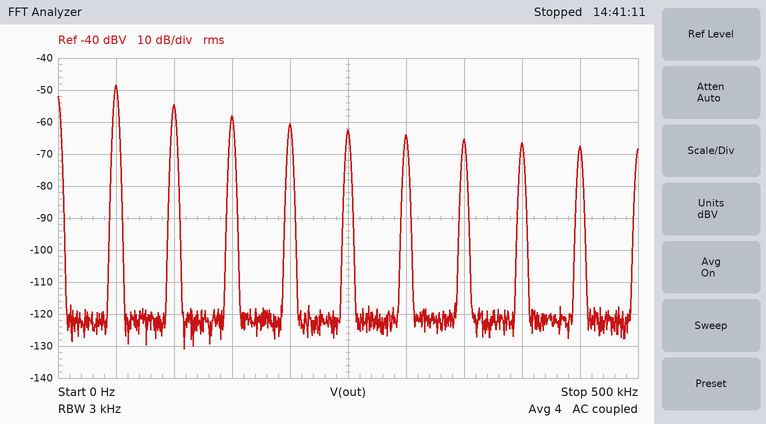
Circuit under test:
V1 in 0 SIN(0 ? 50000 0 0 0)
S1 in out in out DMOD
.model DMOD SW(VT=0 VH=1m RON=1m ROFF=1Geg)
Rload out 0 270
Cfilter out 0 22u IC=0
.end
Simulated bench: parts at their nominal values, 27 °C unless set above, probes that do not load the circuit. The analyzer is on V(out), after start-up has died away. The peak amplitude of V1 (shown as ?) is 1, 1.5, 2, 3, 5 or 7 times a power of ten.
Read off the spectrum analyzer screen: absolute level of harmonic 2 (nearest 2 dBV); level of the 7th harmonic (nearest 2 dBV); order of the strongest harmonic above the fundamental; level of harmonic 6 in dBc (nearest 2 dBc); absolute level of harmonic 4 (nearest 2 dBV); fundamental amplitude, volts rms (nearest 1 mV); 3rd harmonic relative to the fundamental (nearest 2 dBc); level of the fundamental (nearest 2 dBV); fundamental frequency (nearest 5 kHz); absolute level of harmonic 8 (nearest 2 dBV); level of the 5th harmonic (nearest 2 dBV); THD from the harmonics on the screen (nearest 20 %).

-54 dBV
-66 dBV
2
-16 dBc
-60 dBV
4 mV
-10 dBc
-48 dBV
50 kHz
-66 dBV
-62 dBV
80 %
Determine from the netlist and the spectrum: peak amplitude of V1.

5 V
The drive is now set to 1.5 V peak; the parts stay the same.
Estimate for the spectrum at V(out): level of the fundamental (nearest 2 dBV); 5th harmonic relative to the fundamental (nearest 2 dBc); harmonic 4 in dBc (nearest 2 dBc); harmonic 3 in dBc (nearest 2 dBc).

-58 dBV
-10 dBc
-10 dBc
-8 dBc
